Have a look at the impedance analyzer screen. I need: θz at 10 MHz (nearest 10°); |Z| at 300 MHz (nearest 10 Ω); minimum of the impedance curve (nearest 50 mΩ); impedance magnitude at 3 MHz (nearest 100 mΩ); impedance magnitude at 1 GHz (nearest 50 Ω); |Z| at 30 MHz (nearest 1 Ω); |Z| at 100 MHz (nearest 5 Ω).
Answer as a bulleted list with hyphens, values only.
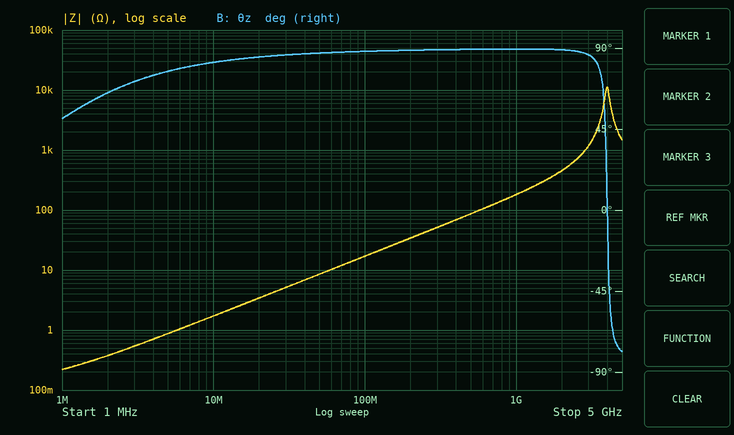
- 80°
- 50 Ω
- 200 mΩ
- 500 mΩ
- 200 Ω
- 5 Ω
- 15 Ω
